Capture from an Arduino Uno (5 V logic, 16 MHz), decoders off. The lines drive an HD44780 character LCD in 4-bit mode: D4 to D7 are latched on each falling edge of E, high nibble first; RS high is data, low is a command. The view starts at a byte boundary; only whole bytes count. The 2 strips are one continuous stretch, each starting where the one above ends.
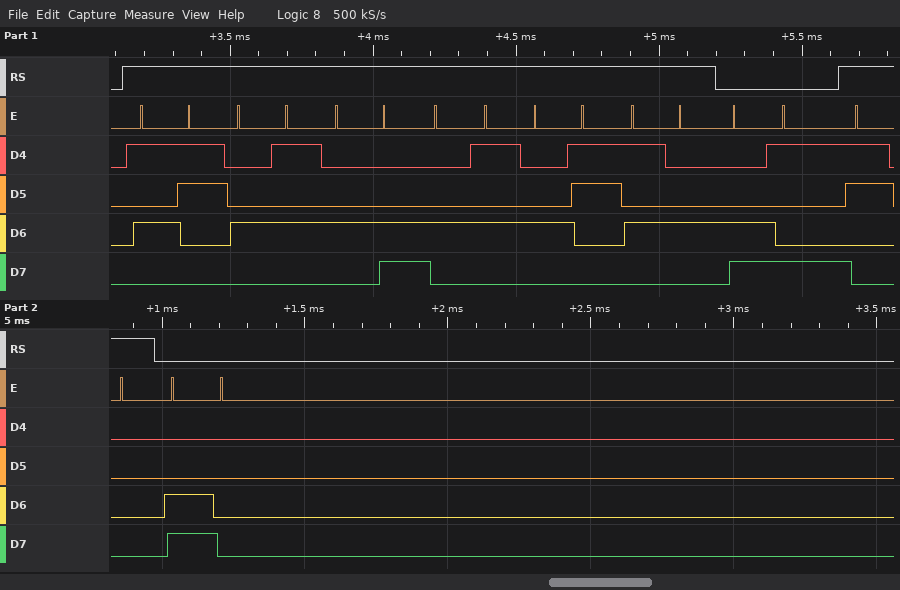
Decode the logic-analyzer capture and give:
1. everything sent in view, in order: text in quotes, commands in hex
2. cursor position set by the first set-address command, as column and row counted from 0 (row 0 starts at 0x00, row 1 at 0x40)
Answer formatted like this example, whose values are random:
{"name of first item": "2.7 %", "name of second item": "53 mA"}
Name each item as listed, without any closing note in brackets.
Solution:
{"everything sent in view, in order: text in quotes, commands in hex": "\"SELECT\" 0xC9 \"0\" 0xC0", "cursor position set by the first set-address command, as column and row counted from 0": "column 9, row 1"}
